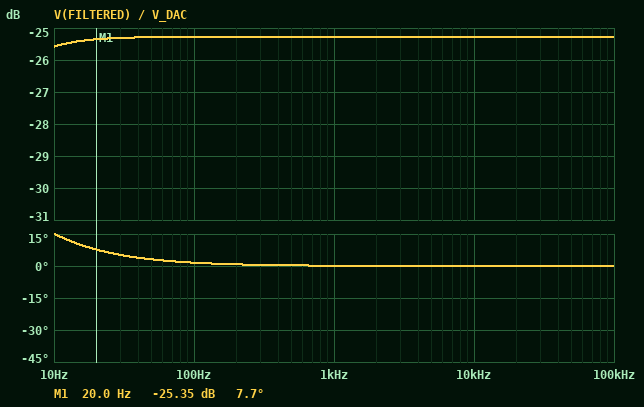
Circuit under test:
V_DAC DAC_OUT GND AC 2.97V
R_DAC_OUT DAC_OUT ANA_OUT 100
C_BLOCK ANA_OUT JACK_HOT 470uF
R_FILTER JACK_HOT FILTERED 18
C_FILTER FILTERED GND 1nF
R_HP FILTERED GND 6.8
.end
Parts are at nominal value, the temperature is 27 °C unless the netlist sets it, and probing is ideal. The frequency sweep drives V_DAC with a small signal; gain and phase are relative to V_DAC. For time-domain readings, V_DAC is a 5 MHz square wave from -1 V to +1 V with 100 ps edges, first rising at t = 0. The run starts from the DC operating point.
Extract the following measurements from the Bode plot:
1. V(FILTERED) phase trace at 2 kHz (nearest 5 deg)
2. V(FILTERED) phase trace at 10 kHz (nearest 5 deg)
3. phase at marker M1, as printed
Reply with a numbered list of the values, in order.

1. 0 deg
2. 0 deg
3. 7.7 deg
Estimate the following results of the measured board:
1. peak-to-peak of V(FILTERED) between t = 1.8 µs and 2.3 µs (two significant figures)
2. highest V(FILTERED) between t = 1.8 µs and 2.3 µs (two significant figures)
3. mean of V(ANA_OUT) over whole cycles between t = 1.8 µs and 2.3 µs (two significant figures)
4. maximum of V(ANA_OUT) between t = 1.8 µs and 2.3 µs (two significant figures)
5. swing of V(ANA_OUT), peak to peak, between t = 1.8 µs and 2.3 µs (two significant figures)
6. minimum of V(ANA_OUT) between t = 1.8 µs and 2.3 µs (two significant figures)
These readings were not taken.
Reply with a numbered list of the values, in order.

1. 110 mV
2. 110 mV
3. -800 mV
4. -600 mV
5. 400 mV
6. -1.0 V
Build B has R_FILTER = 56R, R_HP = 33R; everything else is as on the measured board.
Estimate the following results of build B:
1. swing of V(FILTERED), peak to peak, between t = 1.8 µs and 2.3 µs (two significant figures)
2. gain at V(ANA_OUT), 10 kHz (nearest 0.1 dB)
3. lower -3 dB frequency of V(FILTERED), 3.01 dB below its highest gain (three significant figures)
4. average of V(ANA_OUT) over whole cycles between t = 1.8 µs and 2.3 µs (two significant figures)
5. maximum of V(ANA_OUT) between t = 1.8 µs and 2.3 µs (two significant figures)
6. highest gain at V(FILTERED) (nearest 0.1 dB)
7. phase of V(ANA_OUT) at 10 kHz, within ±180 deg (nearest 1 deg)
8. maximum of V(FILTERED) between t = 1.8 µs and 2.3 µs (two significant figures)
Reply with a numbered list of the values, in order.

1. 330 mV
2. -6.5 dB
3. 1.79 Hz
4. -530 mV
5. -64 mV
6. -15.2 dB
7. 0 deg
8. 340 mV
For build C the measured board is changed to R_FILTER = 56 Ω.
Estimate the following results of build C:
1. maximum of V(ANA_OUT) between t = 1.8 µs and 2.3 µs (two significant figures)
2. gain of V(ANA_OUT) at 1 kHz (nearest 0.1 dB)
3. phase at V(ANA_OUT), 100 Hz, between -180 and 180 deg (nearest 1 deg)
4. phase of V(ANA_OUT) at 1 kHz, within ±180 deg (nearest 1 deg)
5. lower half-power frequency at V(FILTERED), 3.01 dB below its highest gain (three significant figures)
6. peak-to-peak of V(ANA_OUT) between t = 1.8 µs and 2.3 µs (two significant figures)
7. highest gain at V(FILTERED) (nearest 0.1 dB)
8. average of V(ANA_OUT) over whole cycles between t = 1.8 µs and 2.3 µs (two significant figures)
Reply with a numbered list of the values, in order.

1. -230 mV
2. -8.3 dB
3. -2 deg
4. 0 deg
5. 2.08 Hz
6. 770 mV
7. -27.6 dB
8. -610 mV
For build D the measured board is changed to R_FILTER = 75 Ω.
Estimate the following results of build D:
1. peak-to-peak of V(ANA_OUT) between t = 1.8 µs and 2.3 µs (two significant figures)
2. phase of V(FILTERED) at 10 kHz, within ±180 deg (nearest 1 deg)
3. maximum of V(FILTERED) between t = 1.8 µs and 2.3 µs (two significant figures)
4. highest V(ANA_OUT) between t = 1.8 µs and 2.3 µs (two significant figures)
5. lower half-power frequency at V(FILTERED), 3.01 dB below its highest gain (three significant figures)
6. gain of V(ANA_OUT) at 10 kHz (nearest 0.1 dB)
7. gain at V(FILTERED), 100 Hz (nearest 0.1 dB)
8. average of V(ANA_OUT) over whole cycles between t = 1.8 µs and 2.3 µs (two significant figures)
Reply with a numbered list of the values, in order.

1. 900 mV
2. 0 deg
3. 75 mV
4. -100 mV
5. 1.86 Hz
6. -6.9 dB
7. -28.5 dB
8. -550 mV
